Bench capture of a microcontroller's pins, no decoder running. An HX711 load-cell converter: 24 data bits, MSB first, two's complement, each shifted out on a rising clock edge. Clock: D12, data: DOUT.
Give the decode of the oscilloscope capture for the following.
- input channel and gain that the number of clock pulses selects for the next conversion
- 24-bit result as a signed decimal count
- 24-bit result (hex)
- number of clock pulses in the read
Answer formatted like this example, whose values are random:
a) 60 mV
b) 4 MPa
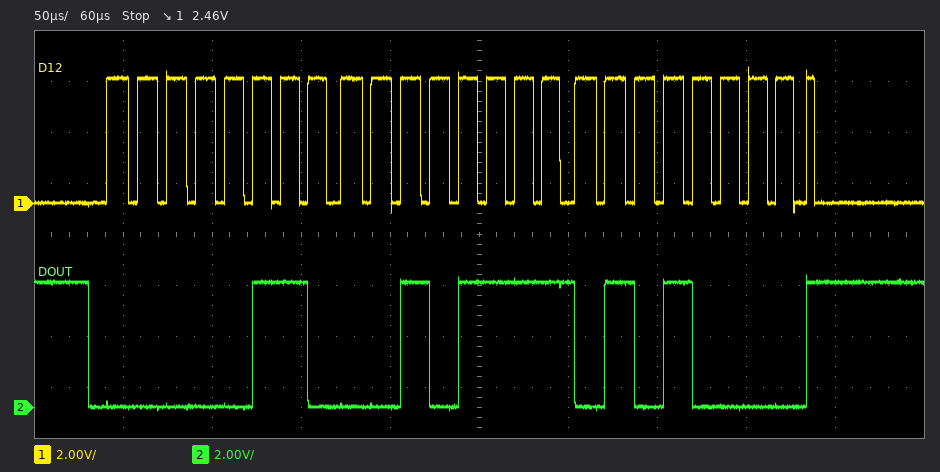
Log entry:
a) channel A, gain 128
b) 405328
c) 0x062F50
d) 25
